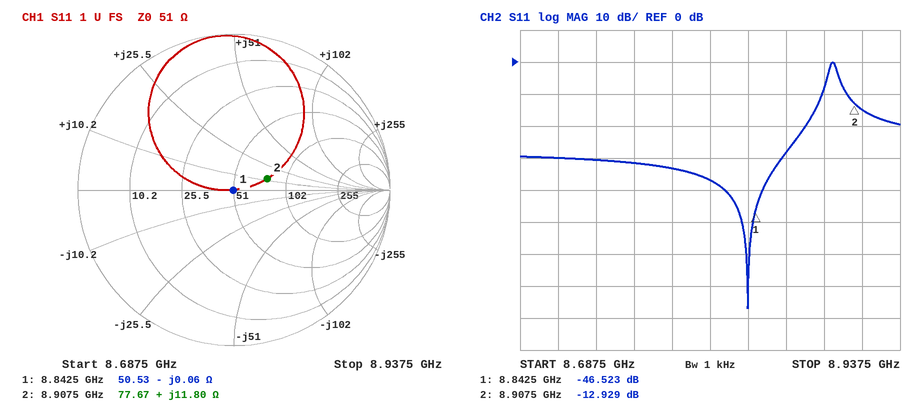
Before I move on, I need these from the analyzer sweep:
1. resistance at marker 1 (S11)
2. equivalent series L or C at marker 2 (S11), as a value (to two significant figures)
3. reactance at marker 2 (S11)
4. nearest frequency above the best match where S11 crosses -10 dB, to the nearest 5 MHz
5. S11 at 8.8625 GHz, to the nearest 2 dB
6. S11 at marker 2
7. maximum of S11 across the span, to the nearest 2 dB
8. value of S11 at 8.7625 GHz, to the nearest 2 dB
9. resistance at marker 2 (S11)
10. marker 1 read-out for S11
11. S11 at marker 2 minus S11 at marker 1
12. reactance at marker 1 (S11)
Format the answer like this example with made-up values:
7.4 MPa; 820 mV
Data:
50.53 Ω; 210 pH; +11.80 Ω; 8.885 GHz; -28 dB; -12.929 dB; 0 dB; -32 dB; 77.67 Ω; -46.523 dB; 33.594 dB; -0.06 Ω
